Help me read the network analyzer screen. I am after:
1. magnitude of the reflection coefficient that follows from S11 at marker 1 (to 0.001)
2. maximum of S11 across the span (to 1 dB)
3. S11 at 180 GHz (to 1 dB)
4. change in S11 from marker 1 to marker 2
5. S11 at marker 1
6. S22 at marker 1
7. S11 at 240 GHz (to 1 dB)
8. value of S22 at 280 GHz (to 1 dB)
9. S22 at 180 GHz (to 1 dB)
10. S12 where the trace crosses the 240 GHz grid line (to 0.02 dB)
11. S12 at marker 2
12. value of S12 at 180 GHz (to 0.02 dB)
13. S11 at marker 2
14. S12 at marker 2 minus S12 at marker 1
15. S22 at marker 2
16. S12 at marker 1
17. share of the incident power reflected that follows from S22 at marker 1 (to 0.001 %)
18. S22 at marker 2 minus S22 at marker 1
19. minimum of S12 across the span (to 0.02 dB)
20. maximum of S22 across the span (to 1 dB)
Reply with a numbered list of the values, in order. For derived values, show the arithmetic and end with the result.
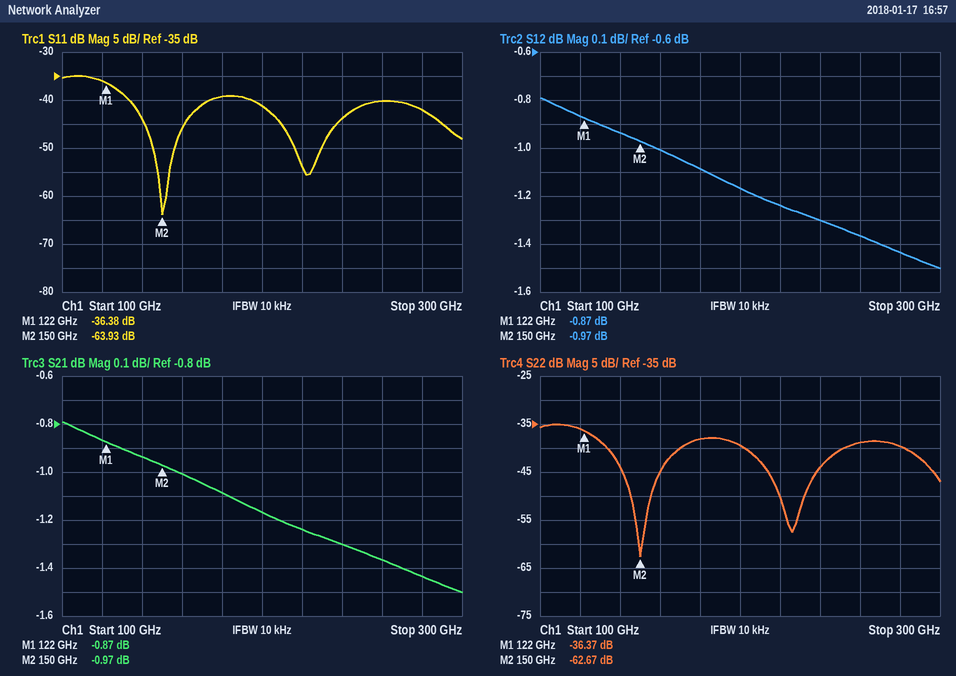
1. 10^(-36.38/20) ≈ 0.015
2. -35 dB
3. -39 dB
4. -63.93 − (-36.38) = -27.55 dB
5. -36.38 dB
6. -36.37 dB
7. -44 dB
8. -40 dB
9. -38 dB
10. -1.30 dB
11. -0.97 dB
12. -1.08 dB
13. -63.93 dB
14. -0.97 − (-0.87) = -0.10 dB
15. -62.67 dB
16. -0.87 dB
17. 10^(-36.37/10) ≈ 0.023 %
18. -62.67 − (-36.37) = -26.30 dB
19. -1.50 dB
20. -35 dB
